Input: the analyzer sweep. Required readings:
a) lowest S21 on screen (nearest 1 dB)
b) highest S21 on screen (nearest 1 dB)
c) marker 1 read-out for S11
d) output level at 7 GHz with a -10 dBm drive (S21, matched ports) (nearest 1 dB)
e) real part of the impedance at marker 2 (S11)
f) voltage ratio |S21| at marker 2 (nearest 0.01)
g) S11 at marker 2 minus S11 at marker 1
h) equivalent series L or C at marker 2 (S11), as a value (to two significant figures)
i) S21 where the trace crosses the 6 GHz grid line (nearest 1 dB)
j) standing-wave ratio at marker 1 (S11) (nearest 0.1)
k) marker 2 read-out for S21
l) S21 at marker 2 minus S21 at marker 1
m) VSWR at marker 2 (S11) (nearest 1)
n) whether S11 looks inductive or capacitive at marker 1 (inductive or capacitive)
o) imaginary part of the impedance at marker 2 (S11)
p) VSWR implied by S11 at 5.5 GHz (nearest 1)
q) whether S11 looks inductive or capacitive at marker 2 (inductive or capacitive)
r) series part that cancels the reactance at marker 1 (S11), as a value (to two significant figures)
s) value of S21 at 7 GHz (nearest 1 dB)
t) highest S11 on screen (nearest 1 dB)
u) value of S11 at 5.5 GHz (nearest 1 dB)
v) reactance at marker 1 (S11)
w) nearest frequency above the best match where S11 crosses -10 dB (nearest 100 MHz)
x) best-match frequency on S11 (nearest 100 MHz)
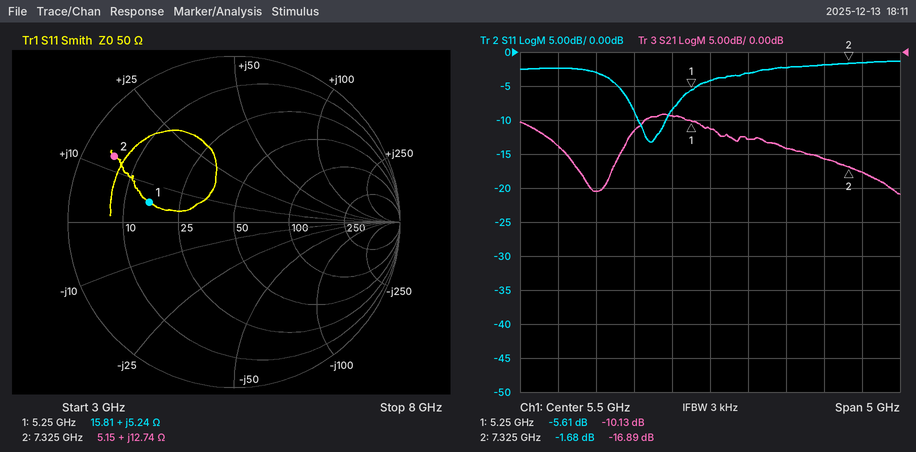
-21 dB
-9 dB
-5.61 dB
-26 dBm
5.15 Ω
0.14
3.93 dB
280 pH
-13 dB
3.2
-16.89 dB
-6.76 dB
10
inductive
+12.74 Ω
4
inductive
5.8 pF
-16 dB
-1 dB
-4 dB
+5.24 Ω
4.9 GHz
4.7 GHz
